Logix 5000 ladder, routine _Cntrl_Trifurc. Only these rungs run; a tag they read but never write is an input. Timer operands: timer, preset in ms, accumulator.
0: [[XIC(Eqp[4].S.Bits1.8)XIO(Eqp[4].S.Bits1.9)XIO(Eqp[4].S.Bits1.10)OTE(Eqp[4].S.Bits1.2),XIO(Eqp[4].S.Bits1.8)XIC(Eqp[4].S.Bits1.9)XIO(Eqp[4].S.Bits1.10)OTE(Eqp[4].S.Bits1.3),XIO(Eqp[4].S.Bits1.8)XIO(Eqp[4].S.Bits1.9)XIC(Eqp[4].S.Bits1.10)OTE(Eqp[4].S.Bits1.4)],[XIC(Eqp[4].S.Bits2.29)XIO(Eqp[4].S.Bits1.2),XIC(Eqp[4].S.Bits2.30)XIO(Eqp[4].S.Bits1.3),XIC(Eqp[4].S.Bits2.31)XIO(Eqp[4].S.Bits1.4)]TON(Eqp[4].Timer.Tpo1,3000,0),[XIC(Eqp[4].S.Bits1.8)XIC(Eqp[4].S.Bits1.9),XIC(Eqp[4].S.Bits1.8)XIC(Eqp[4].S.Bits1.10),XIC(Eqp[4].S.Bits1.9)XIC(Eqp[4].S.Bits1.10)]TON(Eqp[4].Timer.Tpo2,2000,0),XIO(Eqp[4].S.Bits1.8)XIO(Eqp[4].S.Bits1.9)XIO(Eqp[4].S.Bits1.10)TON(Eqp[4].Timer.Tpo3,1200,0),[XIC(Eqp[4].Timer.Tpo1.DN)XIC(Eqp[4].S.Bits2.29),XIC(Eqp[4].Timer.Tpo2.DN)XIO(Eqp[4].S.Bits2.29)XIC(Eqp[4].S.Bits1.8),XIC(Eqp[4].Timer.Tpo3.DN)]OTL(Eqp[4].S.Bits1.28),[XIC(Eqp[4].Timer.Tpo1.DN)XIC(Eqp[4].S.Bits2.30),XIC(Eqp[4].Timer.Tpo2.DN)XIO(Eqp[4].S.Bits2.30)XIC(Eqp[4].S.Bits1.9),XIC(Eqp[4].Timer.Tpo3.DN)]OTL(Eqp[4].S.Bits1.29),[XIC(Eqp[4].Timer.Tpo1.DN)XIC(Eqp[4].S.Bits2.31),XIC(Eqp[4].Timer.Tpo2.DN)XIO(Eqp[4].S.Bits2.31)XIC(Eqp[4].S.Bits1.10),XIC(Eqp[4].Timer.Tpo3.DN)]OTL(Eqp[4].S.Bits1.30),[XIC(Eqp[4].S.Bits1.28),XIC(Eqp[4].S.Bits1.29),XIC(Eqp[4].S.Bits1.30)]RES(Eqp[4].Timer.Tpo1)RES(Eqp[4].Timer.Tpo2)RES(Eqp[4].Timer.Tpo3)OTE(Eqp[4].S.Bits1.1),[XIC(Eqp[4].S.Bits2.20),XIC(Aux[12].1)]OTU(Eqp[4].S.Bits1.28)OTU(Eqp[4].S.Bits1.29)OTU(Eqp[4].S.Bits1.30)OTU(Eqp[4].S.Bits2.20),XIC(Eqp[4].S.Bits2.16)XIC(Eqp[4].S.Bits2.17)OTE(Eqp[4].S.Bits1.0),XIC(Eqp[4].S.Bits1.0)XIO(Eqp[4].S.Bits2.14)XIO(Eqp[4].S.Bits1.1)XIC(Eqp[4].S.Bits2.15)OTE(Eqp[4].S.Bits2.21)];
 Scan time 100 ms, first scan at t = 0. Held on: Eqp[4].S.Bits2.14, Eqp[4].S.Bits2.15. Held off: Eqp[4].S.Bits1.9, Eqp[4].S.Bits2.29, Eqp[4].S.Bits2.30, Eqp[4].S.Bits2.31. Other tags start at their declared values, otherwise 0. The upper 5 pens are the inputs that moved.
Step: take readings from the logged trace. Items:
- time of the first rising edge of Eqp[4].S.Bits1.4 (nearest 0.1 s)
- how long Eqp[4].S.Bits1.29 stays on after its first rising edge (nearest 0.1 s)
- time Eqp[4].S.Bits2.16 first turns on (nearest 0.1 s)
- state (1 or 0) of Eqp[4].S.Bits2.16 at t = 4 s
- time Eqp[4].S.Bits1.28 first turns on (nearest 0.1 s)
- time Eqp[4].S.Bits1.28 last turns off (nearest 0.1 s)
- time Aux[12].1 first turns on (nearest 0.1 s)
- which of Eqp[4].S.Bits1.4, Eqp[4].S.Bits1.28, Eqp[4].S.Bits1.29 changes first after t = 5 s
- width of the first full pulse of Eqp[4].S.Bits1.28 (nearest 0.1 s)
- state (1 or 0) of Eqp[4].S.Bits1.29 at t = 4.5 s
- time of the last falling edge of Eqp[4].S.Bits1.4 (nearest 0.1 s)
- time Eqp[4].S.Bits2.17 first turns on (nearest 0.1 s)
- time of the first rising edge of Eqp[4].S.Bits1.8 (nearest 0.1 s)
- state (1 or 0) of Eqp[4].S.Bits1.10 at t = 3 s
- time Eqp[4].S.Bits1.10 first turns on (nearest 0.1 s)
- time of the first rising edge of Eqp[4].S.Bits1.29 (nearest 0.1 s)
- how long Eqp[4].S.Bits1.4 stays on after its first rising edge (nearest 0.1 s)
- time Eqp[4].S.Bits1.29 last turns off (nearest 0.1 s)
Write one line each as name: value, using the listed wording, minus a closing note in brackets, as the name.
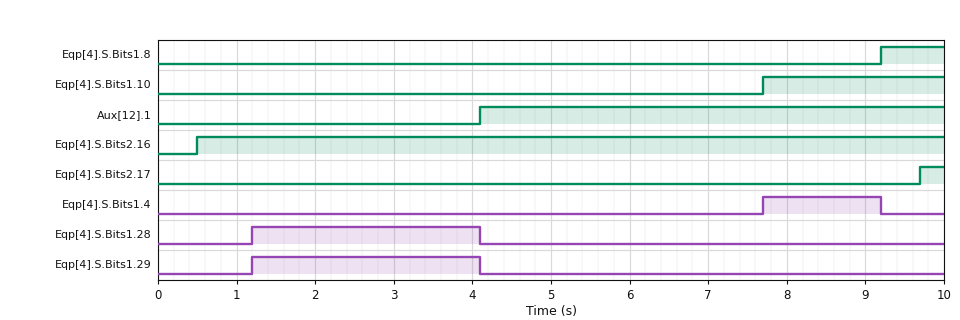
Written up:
time of the first rising edge of Eqp[4].S.Bits1.4: 7.7 s
how long Eqp[4].S.Bits1.29 stays on after its first rising edge: 2.9 s
time Eqp[4].S.Bits2.16 first turns on: 0.5 s
state (1 or 0) of Eqp[4].S.Bits2.16 at t = 4 s: 1
time Eqp[4].S.Bits1.28 first turns on: 1.2 s
time Eqp[4].S.Bits1.28 last turns off: 4.1 s
time Aux[12].1 first turns on: 4.1 s
which of Eqp[4].S.Bits1.4, Eqp[4].S.Bits1.28, Eqp[4].S.Bits1.29 changes first after t = 5 s: Eqp[4].S.Bits1.4
width of the first full pulse of Eqp[4].S.Bits1.28: 2.9 s
state (1 or 0) of Eqp[4].S.Bits1.29 at t = 4.5 s: 0
time of the last falling edge of Eqp[4].S.Bits1.4: 9.2 s
time Eqp[4].S.Bits2.17 first turns on: 9.7 s
time of the first rising edge of Eqp[4].S.Bits1.8: 9.2 s
state (1 or 0) of Eqp[4].S.Bits1.10 at t = 3 s: 0
time Eqp[4].S.Bits1.10 first turns on: 7.7 s
time of the first rising edge of Eqp[4].S.Bits1.29: 1.2 s
how long Eqp[4].S.Bits1.4 stays on after its first rising edge: 1.5 s
time Eqp[4].S.Bits1.29 last turns off: 4.1 s
